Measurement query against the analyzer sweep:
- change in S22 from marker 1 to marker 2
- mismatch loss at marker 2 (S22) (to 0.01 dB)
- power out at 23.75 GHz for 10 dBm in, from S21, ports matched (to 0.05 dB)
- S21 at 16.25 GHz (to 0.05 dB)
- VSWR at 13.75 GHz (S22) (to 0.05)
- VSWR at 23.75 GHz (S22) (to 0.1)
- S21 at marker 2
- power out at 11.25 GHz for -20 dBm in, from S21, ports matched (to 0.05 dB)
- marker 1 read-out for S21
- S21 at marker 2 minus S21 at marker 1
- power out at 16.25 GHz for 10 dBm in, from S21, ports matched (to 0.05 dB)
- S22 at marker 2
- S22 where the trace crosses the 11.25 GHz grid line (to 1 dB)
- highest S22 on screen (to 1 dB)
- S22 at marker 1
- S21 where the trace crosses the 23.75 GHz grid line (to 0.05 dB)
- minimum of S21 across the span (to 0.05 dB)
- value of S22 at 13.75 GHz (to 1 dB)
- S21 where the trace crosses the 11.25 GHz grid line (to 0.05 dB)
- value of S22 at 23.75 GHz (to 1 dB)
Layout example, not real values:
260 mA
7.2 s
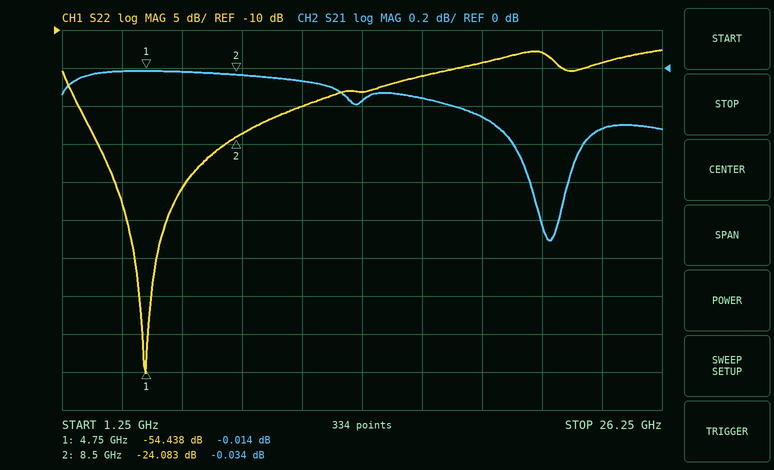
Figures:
30.355 dB
0.02 dB
9.70 dBm
-0.15 dB
1.30
1.5
-0.034 dB
-20.05 dBm
-0.014 dB
-0.020 dB
9.85 dBm
-24.083 dB
-20 dB
-13 dB
-54.438 dB
-0.30 dB
-0.90 dB
-18 dB
-0.05 dB
-14 dB
